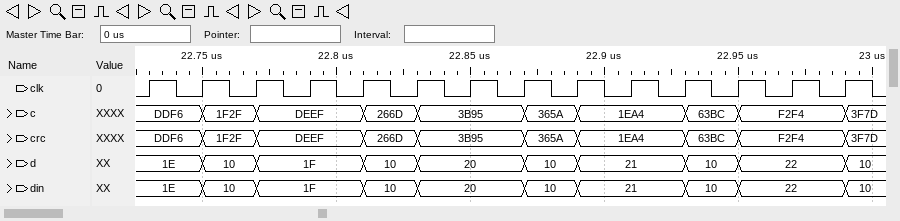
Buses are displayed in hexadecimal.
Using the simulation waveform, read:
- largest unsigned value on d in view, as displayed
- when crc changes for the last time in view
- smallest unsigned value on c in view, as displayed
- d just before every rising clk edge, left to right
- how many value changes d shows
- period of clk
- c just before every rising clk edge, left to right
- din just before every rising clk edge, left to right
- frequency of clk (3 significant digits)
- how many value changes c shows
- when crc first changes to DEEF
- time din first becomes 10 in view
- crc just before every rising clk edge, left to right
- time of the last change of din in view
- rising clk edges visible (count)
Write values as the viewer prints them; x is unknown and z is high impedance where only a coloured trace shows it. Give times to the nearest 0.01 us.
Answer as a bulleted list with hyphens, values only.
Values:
- 22
- 22.99 us
- 1EA4
- 1E, 1E, 10, 1F, 1F, 10, 20, 20, 10, 21, 21, 10, 22, 22
- 9
- 0.02 us
- DDF6, DDF6, 1F2F, DEEF, DEEF, 266D, 3B95, 3B95, 365A, 1EA4, 1EA4, 63BC, F2F4, F2F4
- 1E, 1E, 10, 1F, 1F, 10, 20, 20, 10, 21, 21, 10, 22, 22
- 50.0 MHz
- 9
- 22.77 us
- 22.75 us
- DDF6, DDF6, 1F2F, DEEF, DEEF, 266D, 3B95, 3B95, 365A, 1EA4, 1EA4, 63BC, F2F4, F2F4
- 22.99 us
- 14
